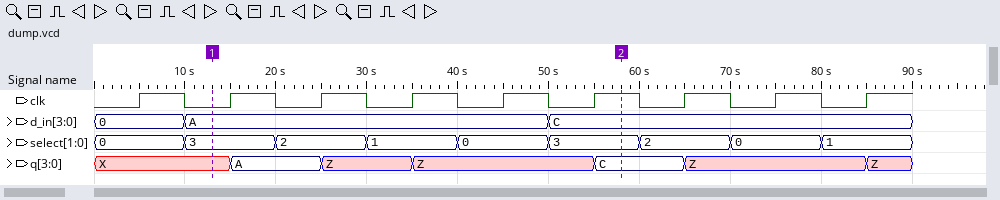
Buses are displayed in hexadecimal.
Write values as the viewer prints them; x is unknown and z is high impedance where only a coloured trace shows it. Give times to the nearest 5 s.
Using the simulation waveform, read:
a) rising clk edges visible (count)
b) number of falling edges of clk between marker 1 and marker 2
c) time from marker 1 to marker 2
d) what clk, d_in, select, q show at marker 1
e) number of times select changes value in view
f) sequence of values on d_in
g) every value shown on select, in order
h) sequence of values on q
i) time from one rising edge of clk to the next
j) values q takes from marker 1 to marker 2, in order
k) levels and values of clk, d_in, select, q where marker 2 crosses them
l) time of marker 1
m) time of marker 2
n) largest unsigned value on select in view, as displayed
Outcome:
9
4
45 s
clk=0, d_in=A, select=3, q=X
8
0, A, C
0, 3, 2, 1, 0, 3, 2, 0, 1
X, A, Z, Z, C, Z, Z
10 s
X, A, Z, Z, C
clk=1, d_in=C, select=3, q=C
15 s
60 s
3
